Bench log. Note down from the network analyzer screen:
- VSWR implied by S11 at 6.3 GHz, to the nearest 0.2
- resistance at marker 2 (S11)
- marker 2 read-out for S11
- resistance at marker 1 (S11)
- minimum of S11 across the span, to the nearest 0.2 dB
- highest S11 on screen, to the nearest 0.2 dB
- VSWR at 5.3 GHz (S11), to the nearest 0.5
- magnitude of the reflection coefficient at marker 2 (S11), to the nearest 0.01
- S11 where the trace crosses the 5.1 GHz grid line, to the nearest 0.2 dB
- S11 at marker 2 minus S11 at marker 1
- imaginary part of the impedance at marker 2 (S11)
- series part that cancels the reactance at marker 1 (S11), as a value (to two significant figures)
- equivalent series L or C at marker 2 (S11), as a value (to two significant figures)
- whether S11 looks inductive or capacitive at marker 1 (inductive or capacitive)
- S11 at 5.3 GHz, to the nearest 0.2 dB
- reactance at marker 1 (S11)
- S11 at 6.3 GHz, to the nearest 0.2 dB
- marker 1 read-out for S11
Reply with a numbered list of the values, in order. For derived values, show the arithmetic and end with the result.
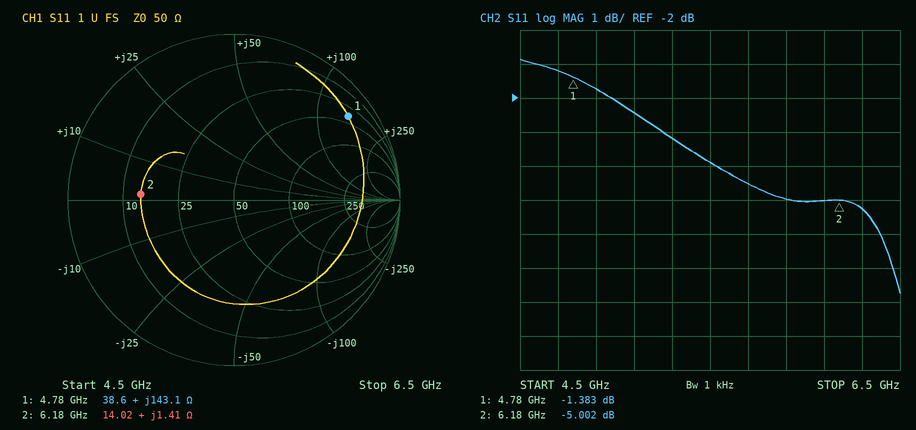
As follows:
1. |Γ| = 10^(-5.2/20) = 0.5495; VSWR = (1 + 0.5495)/(1 − 0.5495) ≈ 3.4
2. 14.02 Ω
3. -5.002 dB
4. 38.6 Ω
5. -7.8 dB
6. -0.8 dB
7. |Γ| = 10^(-3.2/20) = 0.6918; VSWR = (1 + 0.6918)/(1 − 0.6918) ≈ 5.5
8. 0.56
9. -2.4 dB
10. -5.002 − (-1.383) = -3.619 dB
11. +1.41 Ω
12. C = 1/(2π × 4.78 GHz × 143.1 Ω) ≈ 233 fF, so 230 fF to two significant figures
13. L = 1.41 Ω/(2π × 6.18 GHz) ≈ 36 pH
14. inductive
15. -3.2 dB
16. +143.1 Ω
17. -5.2 dB
18. -1.383 dB
